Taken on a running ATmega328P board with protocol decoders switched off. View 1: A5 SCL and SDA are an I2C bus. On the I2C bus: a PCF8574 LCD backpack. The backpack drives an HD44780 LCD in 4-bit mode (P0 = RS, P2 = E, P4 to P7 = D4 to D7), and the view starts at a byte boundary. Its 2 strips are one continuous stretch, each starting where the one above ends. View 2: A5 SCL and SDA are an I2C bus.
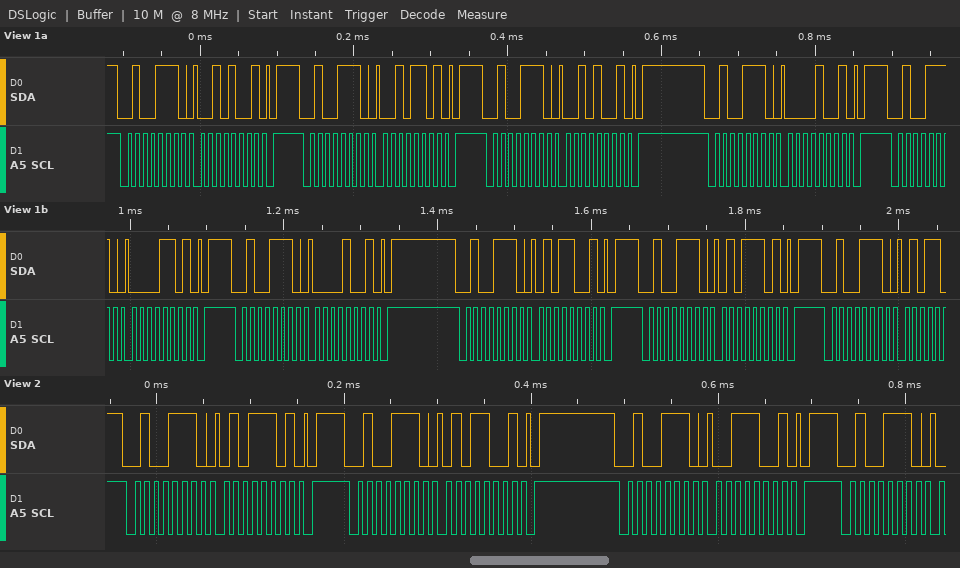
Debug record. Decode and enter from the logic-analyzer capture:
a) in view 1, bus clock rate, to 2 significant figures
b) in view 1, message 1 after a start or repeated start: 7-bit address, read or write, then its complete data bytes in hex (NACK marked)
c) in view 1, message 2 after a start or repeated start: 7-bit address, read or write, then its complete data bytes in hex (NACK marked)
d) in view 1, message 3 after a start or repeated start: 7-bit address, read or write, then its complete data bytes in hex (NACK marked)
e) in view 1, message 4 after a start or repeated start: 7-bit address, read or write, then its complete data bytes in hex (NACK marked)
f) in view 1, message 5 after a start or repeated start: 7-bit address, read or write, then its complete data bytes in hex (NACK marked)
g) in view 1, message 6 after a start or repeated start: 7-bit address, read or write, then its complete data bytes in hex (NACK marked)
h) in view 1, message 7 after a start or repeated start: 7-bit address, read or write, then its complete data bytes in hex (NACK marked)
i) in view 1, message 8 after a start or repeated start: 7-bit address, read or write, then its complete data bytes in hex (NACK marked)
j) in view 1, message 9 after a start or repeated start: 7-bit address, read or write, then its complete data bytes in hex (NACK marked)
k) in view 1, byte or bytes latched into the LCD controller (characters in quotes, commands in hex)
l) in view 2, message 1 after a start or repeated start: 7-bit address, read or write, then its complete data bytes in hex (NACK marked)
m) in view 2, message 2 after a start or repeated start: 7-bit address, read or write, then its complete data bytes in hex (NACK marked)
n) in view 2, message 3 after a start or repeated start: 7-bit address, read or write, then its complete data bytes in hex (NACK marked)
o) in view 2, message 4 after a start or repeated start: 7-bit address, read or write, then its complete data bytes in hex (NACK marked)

100 kHz
0x27 write: 29
0x27 write: 2D
0x27 write: 29
0x27 write: 09
0x27 write: 0D
0x27 write: 09
0x27 write: 59
0x27 write: 5D
0x27 write
' '
0x27 write: 5D
0x27 write: 59
0x27 write: 39
0x27 write
